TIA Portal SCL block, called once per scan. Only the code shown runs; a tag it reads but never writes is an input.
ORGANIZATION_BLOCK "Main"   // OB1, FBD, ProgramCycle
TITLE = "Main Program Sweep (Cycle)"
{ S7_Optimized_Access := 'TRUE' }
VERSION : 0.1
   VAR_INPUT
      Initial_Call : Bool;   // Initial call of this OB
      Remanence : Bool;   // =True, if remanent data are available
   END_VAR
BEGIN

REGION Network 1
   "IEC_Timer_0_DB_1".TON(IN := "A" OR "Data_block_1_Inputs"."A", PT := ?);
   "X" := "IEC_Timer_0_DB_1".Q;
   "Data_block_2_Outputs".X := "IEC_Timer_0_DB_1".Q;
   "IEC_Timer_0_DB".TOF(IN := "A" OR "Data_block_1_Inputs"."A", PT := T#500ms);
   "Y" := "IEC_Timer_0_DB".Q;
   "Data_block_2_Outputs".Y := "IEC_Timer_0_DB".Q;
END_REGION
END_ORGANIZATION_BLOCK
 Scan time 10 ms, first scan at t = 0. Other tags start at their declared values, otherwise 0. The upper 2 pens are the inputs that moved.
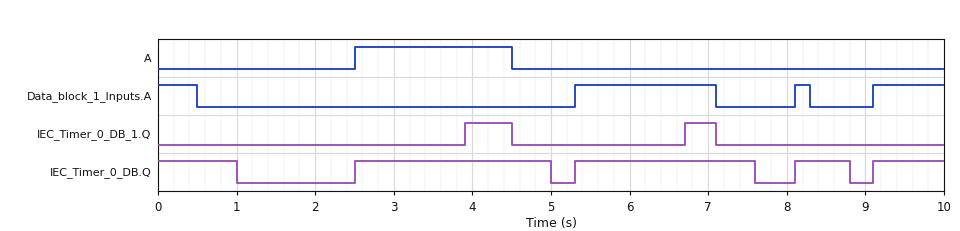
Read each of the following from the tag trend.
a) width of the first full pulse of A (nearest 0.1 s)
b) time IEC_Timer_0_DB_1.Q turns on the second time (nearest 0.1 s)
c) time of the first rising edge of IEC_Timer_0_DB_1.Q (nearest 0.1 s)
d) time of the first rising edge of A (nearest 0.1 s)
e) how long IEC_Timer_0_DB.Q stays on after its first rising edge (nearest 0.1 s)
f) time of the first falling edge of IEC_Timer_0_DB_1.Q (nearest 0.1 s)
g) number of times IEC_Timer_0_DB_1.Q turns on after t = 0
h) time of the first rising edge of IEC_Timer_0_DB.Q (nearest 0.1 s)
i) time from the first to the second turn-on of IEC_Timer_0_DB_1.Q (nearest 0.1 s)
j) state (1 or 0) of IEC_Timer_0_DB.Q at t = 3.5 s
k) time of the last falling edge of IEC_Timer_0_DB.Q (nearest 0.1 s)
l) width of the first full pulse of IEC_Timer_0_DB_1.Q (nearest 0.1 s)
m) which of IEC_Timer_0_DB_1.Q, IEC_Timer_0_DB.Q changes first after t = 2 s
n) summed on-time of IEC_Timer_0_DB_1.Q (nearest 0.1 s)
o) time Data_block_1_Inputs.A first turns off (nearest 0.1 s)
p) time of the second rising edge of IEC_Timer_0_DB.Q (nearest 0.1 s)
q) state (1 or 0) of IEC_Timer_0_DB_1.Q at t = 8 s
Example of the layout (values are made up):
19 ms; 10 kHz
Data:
2.0 s; 6.7 s; 3.9 s; 2.5 s; 2.5 s; 4.5 s; 2; 2.5 s; 2.8 s; 1; 8.8 s; 0.6 s; IEC_Timer_0_DB.Q; 1.0 s; 0.5 s; 5.3 s; 0
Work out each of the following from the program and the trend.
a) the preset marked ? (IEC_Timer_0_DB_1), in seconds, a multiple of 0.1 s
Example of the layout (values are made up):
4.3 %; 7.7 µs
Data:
1.4 s
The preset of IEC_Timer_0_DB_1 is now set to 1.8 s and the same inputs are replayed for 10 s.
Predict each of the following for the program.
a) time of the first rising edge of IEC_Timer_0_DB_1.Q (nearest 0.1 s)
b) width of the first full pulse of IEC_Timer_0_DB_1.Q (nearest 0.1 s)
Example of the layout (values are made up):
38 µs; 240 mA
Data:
4.3 s; 0.2 s
